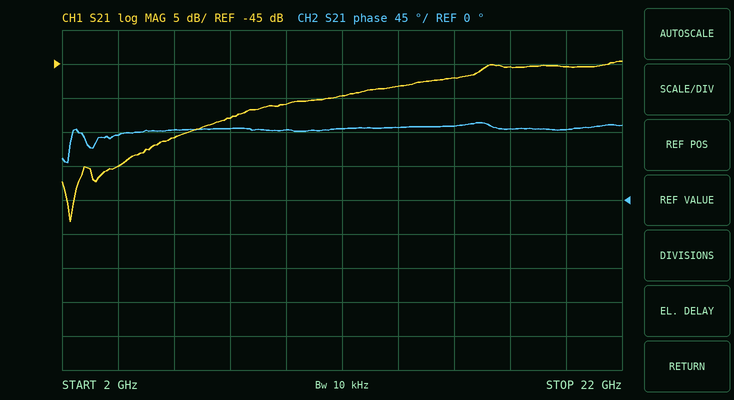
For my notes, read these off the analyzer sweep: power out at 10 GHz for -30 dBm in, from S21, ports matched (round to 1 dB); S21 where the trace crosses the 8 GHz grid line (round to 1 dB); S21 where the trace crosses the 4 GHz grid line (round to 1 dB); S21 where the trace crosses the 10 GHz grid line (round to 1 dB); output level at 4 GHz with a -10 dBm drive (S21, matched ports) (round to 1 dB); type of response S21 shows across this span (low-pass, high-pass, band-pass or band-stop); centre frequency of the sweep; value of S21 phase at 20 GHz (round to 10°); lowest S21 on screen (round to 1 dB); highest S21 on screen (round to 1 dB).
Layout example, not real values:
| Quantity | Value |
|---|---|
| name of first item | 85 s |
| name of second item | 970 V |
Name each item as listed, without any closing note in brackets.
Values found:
| Quantity | Value |
|---|---|
| power out at 10 GHz for -30 dBm in, from S21, ports matched | -81 dBm |
| S21 where the trace crosses the 8 GHz grid line | -53 dB |
| S21 where the trace crosses the 4 GHz grid line | -60 dB |
| S21 where the trace crosses the 10 GHz grid line | -51 dB |
| output level at 4 GHz with a -10 dBm drive (S21, matched ports) | -70 dBm |
| type of response S21 shows across this span | high-pass |
| centre frequency of the sweep | 12 GHz |
| value of S21 phase at 20 GHz | 90° |
| lowest S21 on screen | -68 dB |
| highest S21 on screen | -45 dB |
